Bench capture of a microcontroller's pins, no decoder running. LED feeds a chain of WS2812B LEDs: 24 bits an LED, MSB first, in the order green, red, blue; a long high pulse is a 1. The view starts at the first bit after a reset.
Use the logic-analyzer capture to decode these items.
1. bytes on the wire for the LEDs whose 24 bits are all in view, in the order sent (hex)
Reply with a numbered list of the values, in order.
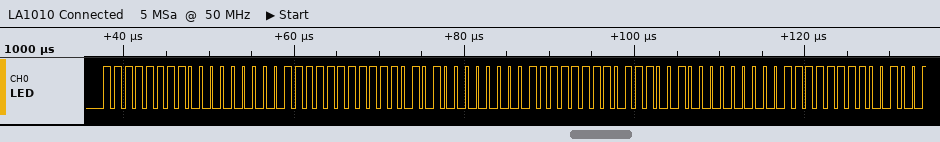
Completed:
1. FF 00 7F F5 00 FF 72 00 FF
